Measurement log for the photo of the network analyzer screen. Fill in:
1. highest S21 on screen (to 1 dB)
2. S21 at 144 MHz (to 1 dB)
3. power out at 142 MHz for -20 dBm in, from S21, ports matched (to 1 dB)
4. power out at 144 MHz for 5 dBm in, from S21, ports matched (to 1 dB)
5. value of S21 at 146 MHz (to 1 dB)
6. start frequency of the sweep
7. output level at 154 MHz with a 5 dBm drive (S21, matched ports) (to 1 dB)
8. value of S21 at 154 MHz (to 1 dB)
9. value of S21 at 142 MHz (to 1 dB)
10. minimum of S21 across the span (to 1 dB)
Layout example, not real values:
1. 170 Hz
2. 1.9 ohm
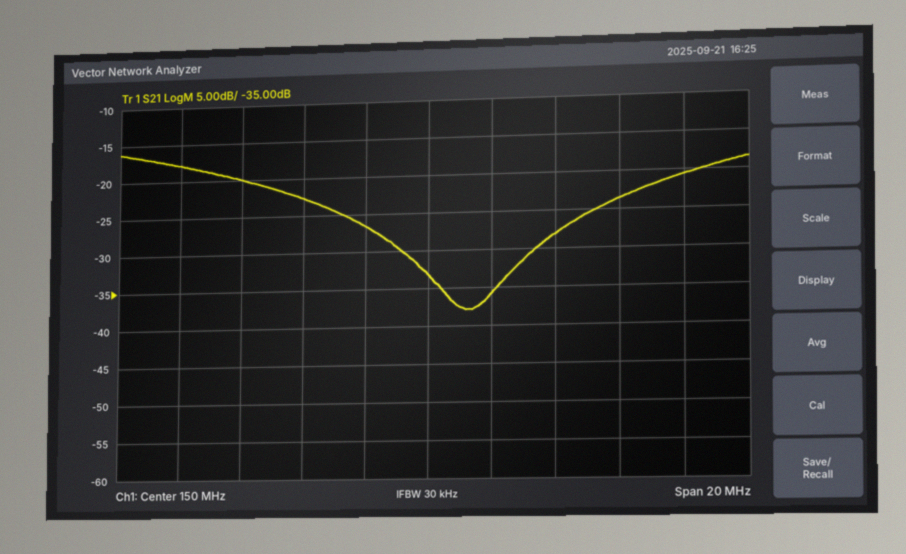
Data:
1. -16 dB
2. -20 dB
3. -38 dBm
4. -15 dBm
5. -23 dB
6. 140 MHz
7. -23 dBm
8. -28 dB
9. -18 dB
10. -38 dB
